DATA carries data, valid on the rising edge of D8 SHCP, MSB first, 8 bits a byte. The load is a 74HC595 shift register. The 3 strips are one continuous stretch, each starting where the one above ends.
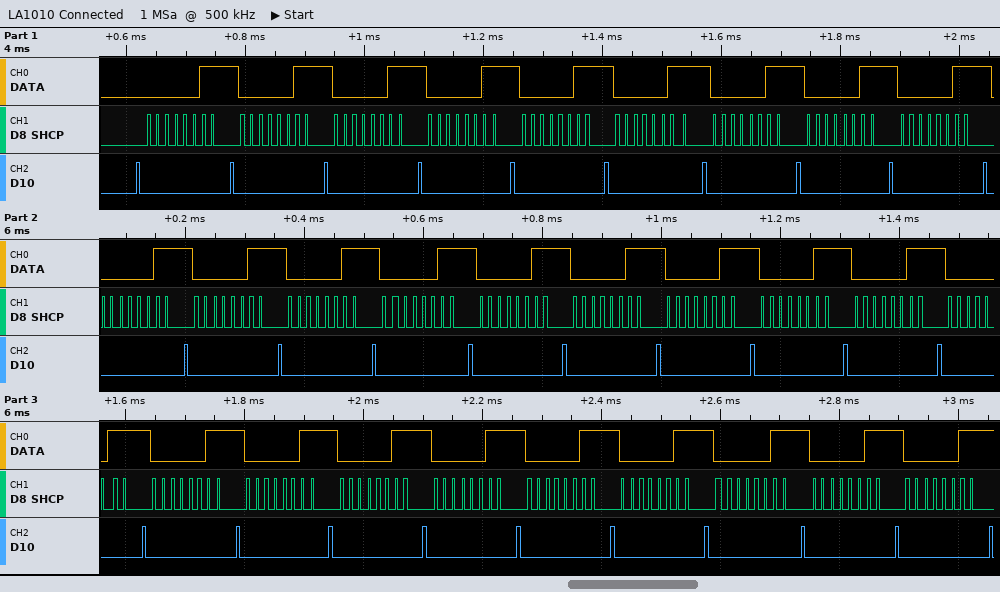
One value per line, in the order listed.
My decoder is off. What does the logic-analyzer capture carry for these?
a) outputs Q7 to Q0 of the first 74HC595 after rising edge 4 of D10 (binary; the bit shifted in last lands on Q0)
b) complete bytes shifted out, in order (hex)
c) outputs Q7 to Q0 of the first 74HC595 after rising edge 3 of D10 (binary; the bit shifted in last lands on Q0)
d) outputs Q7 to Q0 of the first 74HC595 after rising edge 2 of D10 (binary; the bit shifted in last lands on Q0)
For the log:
00000011
03 03 03 03 03 03 03 03 03 03 03 03 03 03 03 03 03 03 03 03 03 03 03 03 03 03 03 03
00000011
00000011
